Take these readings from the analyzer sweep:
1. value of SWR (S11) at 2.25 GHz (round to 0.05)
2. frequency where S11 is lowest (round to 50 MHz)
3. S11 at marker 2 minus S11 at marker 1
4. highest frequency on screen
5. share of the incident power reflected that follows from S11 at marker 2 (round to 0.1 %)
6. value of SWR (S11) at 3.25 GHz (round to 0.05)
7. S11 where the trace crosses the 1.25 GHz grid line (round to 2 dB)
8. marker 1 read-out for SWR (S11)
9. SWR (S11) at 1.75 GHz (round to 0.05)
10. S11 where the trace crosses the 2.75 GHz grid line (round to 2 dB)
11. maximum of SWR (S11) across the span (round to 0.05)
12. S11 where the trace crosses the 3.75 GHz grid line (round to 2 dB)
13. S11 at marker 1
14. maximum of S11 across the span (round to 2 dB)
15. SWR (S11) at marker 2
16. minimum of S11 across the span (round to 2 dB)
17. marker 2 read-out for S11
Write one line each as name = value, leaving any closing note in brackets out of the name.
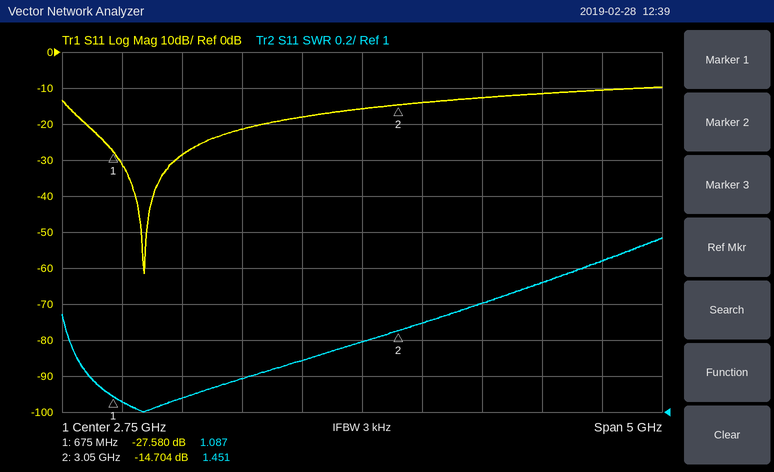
value of SWR (S11) at 2.25 GHz = 1.30
frequency where S11 is lowest = 950 MHz
S11 at marker 2 minus S11 at marker 1 = 12.876 dB
highest frequency on screen = 5.25 GHz
share of the incident power reflected that follows from S11 at marker 2 = 3.4 %
value of SWR (S11) at 3.25 GHz = 1.50
S11 where the trace crosses the 1.25 GHz grid line = -28 dB
marker 1 read-out for SWR = 1.087
SWR (S11) at 1.75 GHz = 1.20
S11 where the trace crosses the 2.75 GHz grid line = -16 dB
maximum of SWR (S11) across the span = 1.95
S11 where the trace crosses the 3.75 GHz grid line = -12 dB
S11 at marker 1 = -27.580 dB
maximum of S11 across the span = -10 dB
SWR (S11) at marker 2 = 1.451
minimum of S11 across the span = -62 dB
marker 2 read-out for S11 = -14.704 dB
